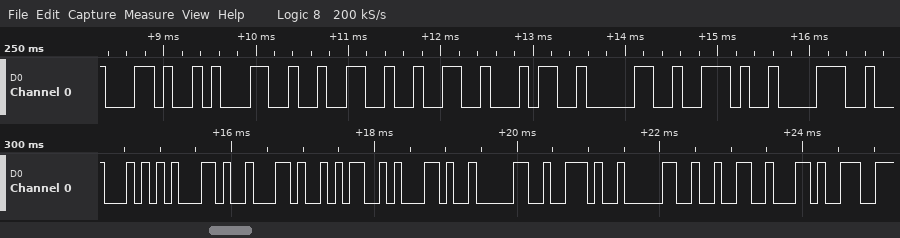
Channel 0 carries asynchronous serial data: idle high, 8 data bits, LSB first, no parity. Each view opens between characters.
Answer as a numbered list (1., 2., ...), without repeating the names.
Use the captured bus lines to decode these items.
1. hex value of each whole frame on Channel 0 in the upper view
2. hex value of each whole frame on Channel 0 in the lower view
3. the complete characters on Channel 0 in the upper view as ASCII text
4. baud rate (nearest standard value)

1. 2C, 31, 32, 32, 34, 30, 2E, 38
2. 54, 2C, 2C, 4D, 2C, 30, 2E, 30, 32, 2C
3. ",12240.8"
4. 9600 baud
